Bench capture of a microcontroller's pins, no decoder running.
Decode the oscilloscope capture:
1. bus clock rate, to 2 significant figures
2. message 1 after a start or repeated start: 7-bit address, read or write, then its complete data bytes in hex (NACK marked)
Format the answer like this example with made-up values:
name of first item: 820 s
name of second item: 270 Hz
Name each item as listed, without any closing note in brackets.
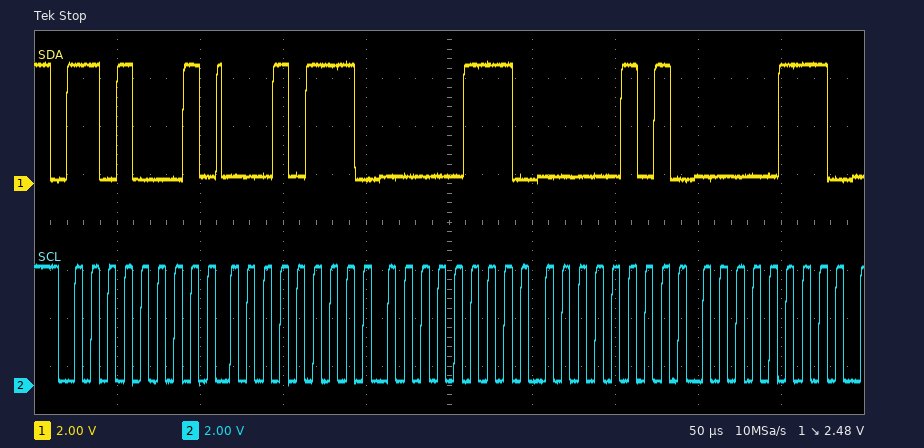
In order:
bus clock rate, to 2 significant figures: 100 kHz
message 1 after a start or repeated start: 7-bit address, read or write, then its complete data bytes in hex: 0x68 read: 17 07 05 07
